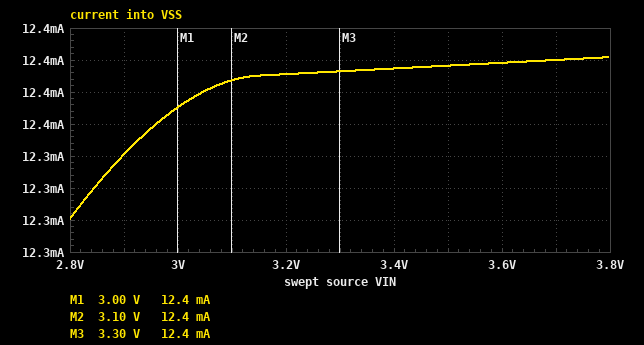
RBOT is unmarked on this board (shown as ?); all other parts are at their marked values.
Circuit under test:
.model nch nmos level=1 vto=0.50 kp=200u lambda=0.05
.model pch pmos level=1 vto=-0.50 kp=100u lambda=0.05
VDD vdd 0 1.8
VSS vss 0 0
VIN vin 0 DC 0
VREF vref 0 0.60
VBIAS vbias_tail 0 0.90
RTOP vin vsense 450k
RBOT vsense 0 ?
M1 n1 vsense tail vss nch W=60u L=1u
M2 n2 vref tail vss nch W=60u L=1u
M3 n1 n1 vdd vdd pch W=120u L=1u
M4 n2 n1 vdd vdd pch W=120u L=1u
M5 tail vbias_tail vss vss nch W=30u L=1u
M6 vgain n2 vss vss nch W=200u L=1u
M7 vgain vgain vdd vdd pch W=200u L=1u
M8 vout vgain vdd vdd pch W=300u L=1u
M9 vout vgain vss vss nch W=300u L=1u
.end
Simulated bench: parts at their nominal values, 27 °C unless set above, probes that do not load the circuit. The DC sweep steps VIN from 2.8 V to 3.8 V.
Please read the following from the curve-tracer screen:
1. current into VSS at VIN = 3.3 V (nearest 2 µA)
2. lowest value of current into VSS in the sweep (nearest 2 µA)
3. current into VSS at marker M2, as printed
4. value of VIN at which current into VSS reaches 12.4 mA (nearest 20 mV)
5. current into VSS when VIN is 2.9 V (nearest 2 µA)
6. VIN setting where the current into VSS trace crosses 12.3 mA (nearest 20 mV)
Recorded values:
12.376 mA
12.330 mA
12.4 mA
3.04 V
12.350 mA
2.84 V
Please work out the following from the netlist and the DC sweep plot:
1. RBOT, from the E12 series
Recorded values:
270 kΩ
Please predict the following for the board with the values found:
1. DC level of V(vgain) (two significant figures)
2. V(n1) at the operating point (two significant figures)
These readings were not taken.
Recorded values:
1.3 V
1.3 V
